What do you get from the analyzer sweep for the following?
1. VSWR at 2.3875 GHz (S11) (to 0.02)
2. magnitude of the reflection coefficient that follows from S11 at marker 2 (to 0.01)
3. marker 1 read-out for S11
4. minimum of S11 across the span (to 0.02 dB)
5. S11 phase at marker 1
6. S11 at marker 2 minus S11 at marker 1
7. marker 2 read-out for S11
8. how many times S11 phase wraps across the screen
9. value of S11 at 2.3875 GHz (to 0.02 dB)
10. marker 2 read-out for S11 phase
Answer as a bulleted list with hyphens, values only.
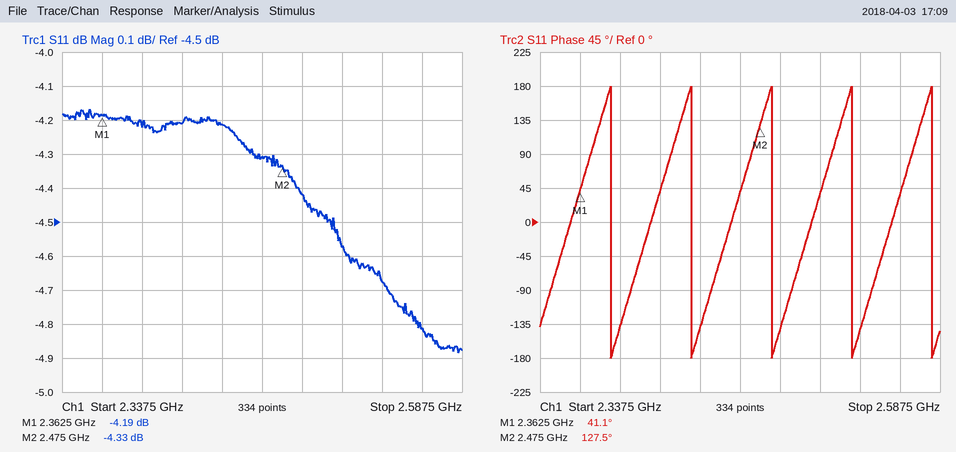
- 4.20
- 0.61
- -4.19 dB
- -4.88 dB
- 41.1°
- -0.14 dB
- -4.33 dB
- 5
- -4.22 dB
- 127.5°
